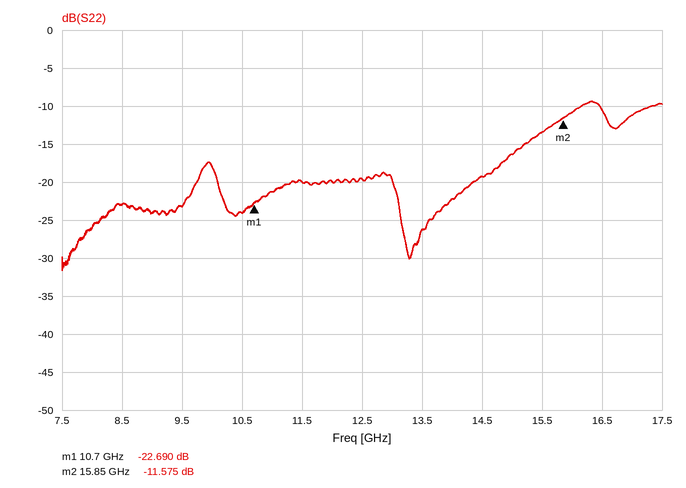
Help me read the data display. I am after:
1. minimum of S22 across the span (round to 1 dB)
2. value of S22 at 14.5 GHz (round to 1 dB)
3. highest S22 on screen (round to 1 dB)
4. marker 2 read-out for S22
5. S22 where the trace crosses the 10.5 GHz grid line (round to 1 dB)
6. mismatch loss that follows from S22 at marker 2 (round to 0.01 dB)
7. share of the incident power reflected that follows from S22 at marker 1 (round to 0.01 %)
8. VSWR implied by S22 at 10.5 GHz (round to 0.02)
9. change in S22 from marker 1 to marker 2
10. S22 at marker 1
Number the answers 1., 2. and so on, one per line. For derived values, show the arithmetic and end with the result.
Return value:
1. -32 dB
2. -19 dB
3. -9 dB
4. -11.575 dB
5. -24 dB
6. −10 log10(1 − 10^(-11.575/10)) ≈ 0.31 dB
7. 10^(-22.69/10) ≈ 0.54 %
8. |Γ| = 10^(-24/20) = 0.0631; VSWR = (1 + 0.0631)/(1 − 0.0631) ≈ 1.13, so 1.14 to the nearest 0.02
9. -11.575 − (-22.69) = 11.115 dB
10. -22.690 dB
